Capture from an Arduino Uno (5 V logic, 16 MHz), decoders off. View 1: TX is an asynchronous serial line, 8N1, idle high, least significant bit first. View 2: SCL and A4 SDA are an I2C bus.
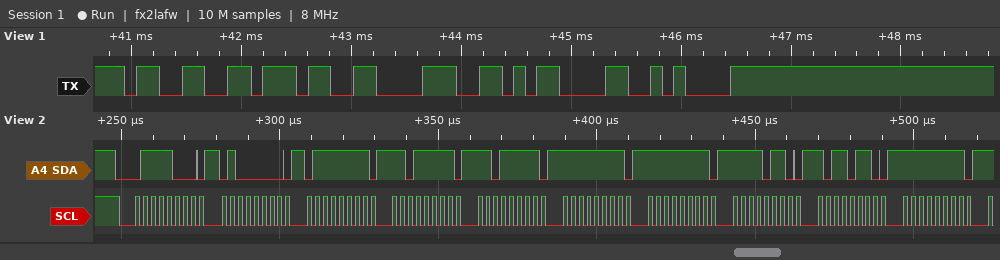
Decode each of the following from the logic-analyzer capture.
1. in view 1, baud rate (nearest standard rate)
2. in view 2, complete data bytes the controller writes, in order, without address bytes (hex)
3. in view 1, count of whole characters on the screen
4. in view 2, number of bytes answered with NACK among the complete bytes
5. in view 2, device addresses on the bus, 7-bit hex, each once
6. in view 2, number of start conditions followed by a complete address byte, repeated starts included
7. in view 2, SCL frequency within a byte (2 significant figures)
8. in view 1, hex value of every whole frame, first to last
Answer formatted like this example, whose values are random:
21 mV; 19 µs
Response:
9600 baud; 40 7F DF DF FF FF F6 B6 FF; 5; 0; 0x3C; 1; 400 kHz; 33 37 38 0D 0A
